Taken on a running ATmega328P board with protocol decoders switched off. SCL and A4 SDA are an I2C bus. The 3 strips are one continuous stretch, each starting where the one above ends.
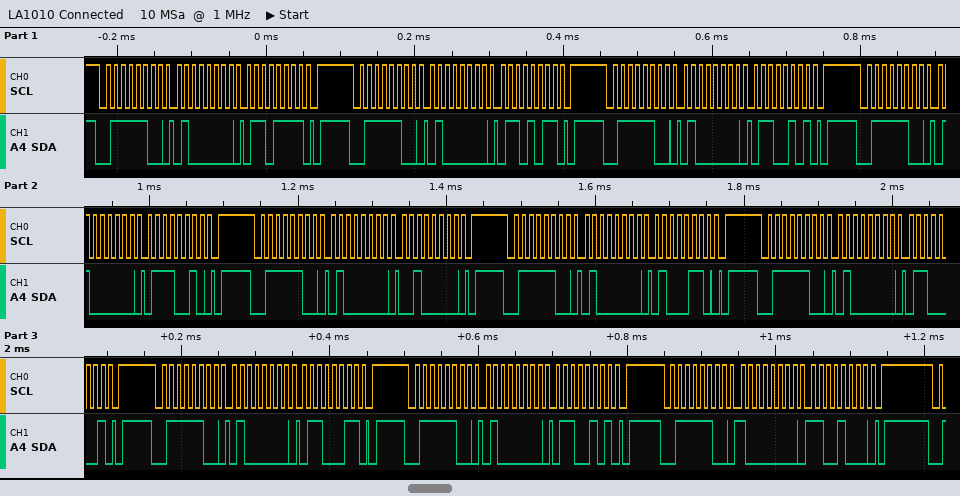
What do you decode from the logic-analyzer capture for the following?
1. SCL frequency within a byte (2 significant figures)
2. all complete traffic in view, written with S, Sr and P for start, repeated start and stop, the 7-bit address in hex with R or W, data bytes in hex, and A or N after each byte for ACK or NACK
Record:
100 kHz
S 3EW A 40 A 6F A P S 3EW A 40 A 6B A P S 3EW A 40 A 65 A P S 3EW A 40 A 72 A P S 3EW A 40 A 20 A P S 3EW A 40 A 46 A P S 3EW A 40 A 61 A P S 3EW A 40 A 63 A P S 3EW A 40 A 65 A P S 3EW A 80 A C8 A P
